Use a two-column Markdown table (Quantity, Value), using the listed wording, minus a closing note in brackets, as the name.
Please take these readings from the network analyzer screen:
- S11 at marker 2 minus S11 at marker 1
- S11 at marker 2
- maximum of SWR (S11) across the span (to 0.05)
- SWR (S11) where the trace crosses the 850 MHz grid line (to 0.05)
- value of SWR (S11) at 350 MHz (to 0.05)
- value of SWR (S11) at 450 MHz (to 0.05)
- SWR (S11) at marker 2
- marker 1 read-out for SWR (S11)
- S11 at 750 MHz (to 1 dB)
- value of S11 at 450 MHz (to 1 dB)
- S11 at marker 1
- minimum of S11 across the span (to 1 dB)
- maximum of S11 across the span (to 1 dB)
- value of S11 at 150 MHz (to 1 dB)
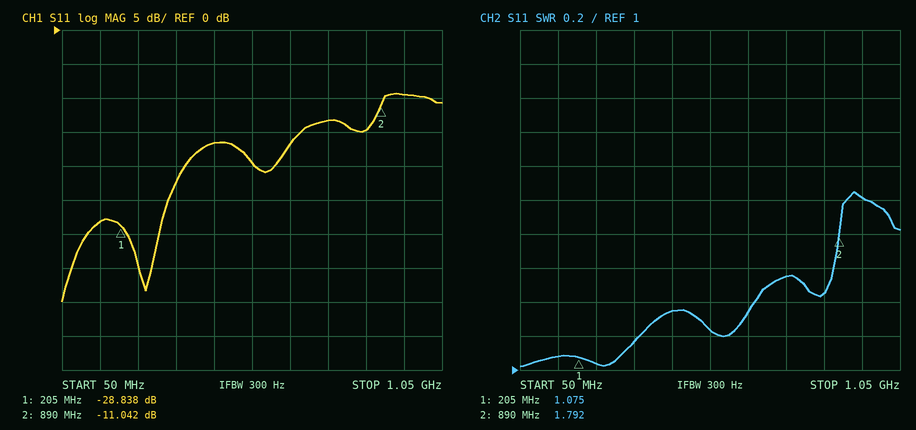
| Quantity | Value |
|---|---|
| S11 at marker 2 minus S11 at marker 1 | 17.796 dB |
| S11 at marker 2 | -11.042 dB |
| maximum of SWR (S11) across the span | 2.05 |
| SWR (S11) where the trace crosses the 850 MHz grid line | 1.45 |
| value of SWR (S11) at 350 MHz | 1.15 |
| value of SWR (S11) at 450 MHz | 1.35 |
| SWR (S11) at marker 2 | 1.792 |
| marker 1 read-out for SWR | 1.075 |
| S11 at 750 MHz | -13 dB |
| value of S11 at 450 MHz | -17 dB |
| S11 at marker 1 | -28.838 dB |
| minimum of S11 across the span | -40 dB |
| maximum of S11 across the span | -9 dB |
| value of S11 at 150 MHz | -28 dB |
